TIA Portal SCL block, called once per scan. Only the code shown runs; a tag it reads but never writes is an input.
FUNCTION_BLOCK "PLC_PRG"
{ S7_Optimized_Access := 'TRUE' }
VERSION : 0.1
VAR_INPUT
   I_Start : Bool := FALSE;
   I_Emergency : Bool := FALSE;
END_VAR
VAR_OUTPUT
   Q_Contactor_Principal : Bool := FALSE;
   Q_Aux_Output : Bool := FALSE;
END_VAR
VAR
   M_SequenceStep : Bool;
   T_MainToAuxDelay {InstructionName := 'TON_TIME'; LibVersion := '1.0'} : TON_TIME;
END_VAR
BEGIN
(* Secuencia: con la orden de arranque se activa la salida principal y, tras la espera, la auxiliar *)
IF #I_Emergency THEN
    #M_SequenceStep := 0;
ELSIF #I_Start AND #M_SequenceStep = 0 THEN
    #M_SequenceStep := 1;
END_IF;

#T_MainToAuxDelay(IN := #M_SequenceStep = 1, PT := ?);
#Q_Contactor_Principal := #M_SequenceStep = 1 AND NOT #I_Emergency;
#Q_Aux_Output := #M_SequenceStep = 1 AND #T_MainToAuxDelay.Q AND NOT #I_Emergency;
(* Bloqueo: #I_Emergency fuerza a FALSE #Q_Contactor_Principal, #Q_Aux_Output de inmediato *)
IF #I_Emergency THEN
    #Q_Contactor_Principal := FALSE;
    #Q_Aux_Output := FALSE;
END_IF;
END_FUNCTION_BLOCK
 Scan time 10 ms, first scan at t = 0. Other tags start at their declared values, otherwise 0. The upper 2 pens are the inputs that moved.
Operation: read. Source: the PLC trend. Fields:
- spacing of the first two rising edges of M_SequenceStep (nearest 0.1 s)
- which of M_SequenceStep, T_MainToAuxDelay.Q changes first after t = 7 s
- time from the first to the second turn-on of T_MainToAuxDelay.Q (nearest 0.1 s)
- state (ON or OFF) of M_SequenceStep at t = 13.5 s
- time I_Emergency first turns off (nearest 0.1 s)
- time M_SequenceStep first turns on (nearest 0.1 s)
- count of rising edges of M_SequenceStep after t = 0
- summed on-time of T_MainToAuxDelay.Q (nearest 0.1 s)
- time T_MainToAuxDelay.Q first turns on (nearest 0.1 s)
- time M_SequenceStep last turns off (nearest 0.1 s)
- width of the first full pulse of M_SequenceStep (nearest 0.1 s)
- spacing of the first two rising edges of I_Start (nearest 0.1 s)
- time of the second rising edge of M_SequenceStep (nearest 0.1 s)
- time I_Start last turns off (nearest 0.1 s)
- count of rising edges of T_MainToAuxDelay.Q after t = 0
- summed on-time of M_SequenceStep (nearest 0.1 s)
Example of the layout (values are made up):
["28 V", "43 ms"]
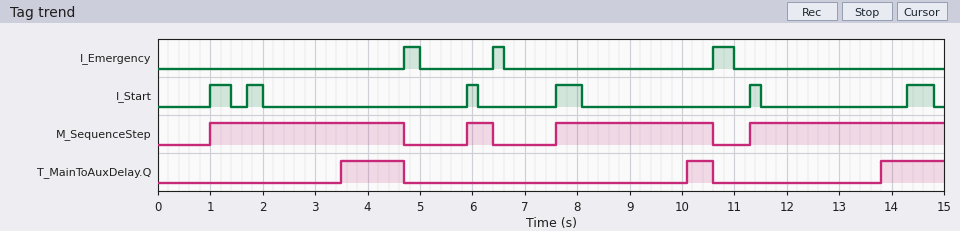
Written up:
["4.9 s", "M_SequenceStep", "6.6 s", "ON", "5.0 s", "1.0 s", "4", "2.9 s", "3.5 s", "10.6 s", "3.7 s", "0.7 s", "5.9 s", "14.8 s", "3", "10.9 s"]
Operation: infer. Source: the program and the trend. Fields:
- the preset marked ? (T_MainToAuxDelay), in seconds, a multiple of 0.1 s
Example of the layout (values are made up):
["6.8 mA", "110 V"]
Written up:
["2.5 s"]
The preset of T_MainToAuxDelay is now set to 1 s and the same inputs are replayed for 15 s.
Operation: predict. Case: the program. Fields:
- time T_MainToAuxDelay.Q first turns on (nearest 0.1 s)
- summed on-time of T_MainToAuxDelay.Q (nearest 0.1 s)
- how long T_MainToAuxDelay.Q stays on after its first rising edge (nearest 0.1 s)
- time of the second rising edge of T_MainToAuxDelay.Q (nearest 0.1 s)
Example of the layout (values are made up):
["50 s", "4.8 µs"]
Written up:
["2.0 s", "7.4 s", "2.7 s", "8.6 s"]
